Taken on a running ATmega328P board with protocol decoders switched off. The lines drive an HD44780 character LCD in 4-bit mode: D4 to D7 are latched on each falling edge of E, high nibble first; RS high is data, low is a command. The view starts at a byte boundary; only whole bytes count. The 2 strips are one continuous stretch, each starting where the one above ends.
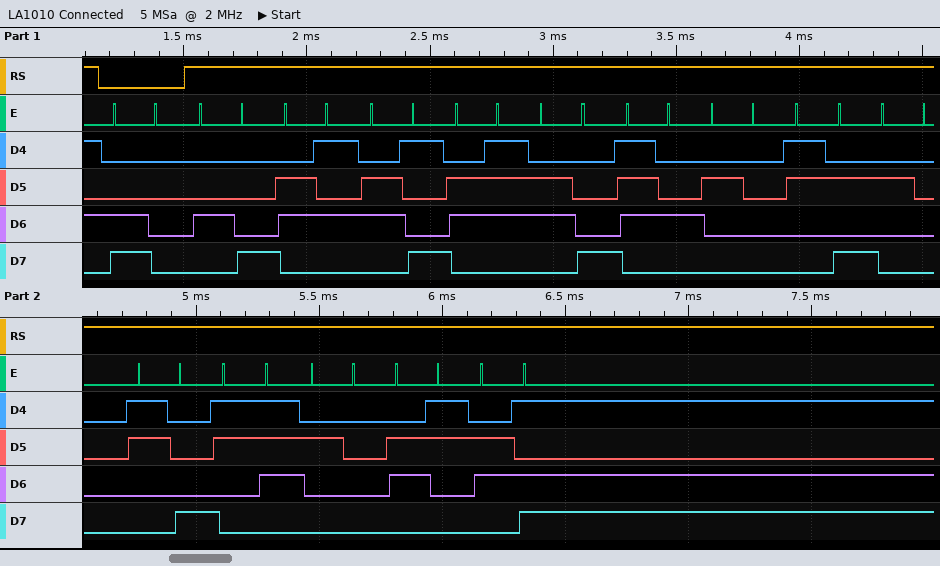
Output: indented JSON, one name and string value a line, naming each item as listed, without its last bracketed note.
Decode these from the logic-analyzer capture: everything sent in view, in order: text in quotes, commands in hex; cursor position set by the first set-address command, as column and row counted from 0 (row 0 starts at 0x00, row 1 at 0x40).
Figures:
{
  "everything sent in view, in order: text in quotes, commands in hex": "0xC0 \"Height : 87 cm\"",
  "cursor position set by the first set-address command, as column and row counted from 0": "column 0, row 1"
}
